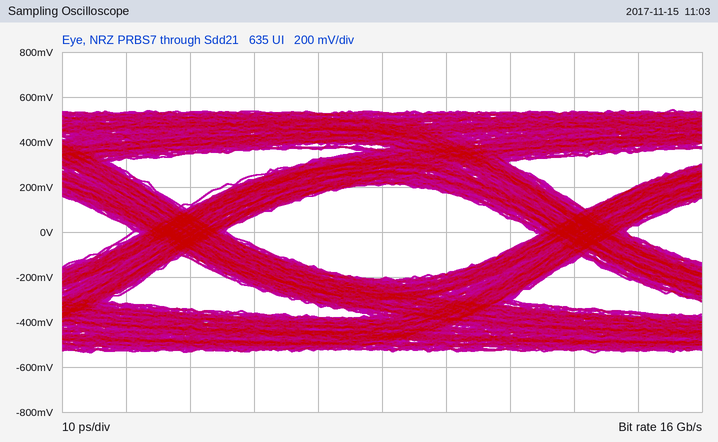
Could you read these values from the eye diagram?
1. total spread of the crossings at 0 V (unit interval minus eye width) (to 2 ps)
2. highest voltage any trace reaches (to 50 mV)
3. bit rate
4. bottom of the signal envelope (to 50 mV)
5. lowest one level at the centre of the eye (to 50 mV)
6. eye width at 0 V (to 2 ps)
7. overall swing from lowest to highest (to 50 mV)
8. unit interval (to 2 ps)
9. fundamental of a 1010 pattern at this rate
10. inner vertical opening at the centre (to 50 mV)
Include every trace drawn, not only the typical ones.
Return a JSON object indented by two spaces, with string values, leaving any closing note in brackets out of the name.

{
  "total spread of the crossings at 0 V (unit interval minus eye width)": "14 ps",
  "highest voltage any trace reaches": "550 mV",
  "bit rate": "16 Gb/s",
  "bottom of the signal envelope": "-550 mV",
  "lowest one level at the centre of the eye": "200 mV",
  "eye width at 0 V": "48 ps",
  "overall swing from lowest to highest": "1.10 V",
  "unit interval": "62 ps",
  "fundamental of a 1010 pattern at this rate": "8 GHz",
  "inner vertical opening at the centre": "400 mV"
}
